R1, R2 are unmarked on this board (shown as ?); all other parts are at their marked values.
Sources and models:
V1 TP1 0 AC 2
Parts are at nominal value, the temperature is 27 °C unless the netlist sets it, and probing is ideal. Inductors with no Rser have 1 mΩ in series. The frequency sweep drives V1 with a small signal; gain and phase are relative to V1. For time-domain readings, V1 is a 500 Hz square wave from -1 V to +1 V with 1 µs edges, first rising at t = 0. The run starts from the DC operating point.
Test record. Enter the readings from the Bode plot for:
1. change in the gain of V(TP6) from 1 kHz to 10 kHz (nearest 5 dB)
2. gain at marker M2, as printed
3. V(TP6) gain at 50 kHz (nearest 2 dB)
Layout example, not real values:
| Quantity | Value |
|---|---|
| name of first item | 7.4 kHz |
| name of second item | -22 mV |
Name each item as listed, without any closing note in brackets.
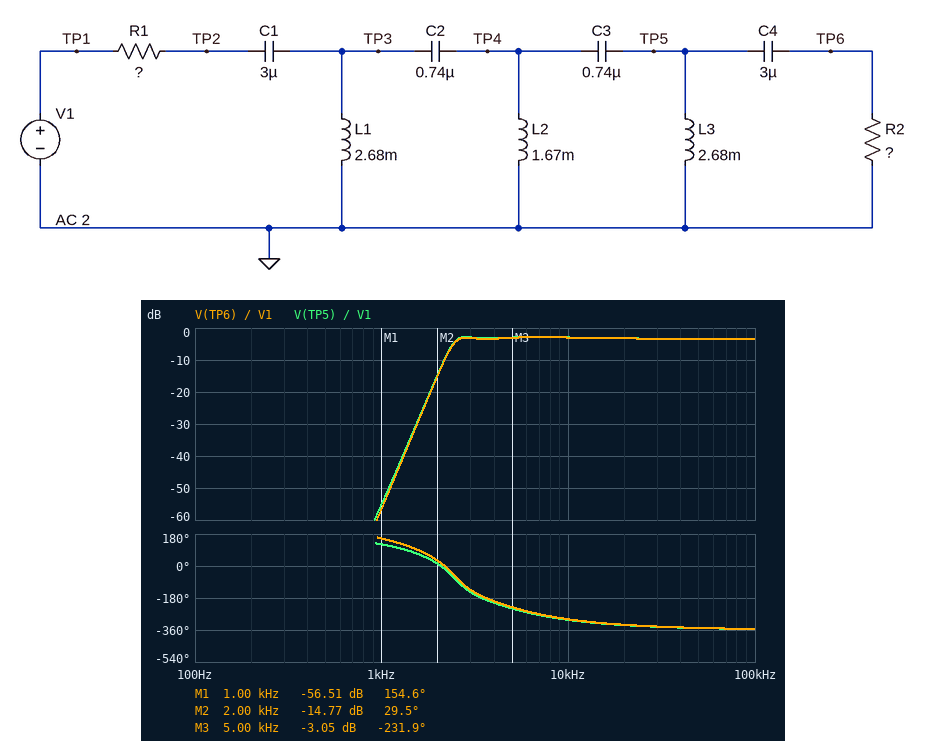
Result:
| Quantity | Value |
|---|---|
| change in the gain of V(TP6) from 1 kHz to 10 kHz | 55 dB |
| gain at marker M2, as printed | -14.77 dB |
| V(TP6) gain at 50 kHz | -4 dB |
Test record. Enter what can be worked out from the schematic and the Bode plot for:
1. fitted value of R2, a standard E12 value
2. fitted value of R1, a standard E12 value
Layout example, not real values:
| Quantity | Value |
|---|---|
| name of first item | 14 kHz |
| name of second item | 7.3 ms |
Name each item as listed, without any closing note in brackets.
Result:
| Quantity | Value |
|---|---|
| fitted value of R2, a standard E12 value | 82 Ω |
| fitted value of R1, a standard E12 value | 39 Ω |
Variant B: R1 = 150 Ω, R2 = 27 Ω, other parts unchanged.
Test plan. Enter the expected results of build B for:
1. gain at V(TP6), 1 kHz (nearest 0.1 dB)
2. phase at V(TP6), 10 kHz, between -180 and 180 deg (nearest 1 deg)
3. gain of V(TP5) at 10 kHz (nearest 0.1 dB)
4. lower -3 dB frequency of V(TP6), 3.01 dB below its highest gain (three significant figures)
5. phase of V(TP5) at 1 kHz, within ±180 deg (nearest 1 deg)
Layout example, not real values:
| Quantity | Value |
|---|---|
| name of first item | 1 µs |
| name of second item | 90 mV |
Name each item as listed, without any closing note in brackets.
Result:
| Quantity | Value |
|---|---|
| gain at V(TP6), 1 kHz | -69.4 dB |
| phase at V(TP6), 10 kHz, between -180 and 180 deg | 54 deg |
| gain of V(TP5) at 10 kHz | -14.3 dB |
| lower -3 dB frequency of V(TP6), 3.01 dB below its highest gain | 2.42 kHz |
| phase of V(TP5) at 1 kHz, within ±180 deg | 92 deg |
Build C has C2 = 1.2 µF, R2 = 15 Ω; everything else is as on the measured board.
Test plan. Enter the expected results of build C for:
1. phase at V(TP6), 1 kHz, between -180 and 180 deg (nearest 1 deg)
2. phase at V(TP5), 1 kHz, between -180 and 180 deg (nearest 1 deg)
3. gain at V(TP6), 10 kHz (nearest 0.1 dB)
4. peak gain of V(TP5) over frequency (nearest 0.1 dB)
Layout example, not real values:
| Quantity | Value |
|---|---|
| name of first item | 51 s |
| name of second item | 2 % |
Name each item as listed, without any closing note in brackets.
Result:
| Quantity | Value |
|---|---|
| phase at V(TP6), 1 kHz, between -180 and 180 deg | -163 deg |
| phase at V(TP5), 1 kHz, between -180 and 180 deg | 123 deg |
| gain at V(TP6), 10 kHz | -11.6 dB |
| peak gain of V(TP5) over frequency | -9.6 dB |
